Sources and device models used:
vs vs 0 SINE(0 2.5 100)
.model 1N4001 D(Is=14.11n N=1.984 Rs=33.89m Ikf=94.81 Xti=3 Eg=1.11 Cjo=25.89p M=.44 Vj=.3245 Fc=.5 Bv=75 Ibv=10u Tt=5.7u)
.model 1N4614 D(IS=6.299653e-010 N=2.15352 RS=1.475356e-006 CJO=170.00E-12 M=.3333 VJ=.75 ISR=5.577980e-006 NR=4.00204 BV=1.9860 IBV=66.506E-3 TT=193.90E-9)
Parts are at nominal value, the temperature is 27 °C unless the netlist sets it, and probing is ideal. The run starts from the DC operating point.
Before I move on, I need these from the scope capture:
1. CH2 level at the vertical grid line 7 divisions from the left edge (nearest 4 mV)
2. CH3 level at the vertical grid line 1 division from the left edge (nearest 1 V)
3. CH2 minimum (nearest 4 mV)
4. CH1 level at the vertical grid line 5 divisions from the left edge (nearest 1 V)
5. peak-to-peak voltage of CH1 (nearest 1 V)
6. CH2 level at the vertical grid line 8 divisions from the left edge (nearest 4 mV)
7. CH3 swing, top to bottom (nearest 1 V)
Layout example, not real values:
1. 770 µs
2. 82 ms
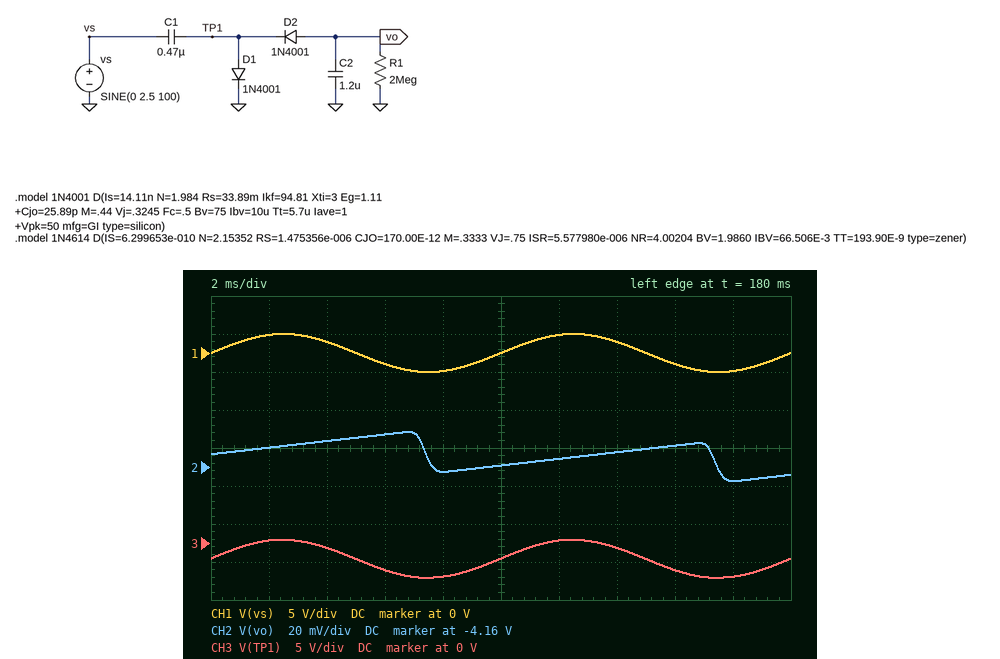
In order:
1. -4.152 V
2. 0 V
3. -4.168 V
4. 0 V
5. 5 V
6. -4.148 V
7. 5 V
